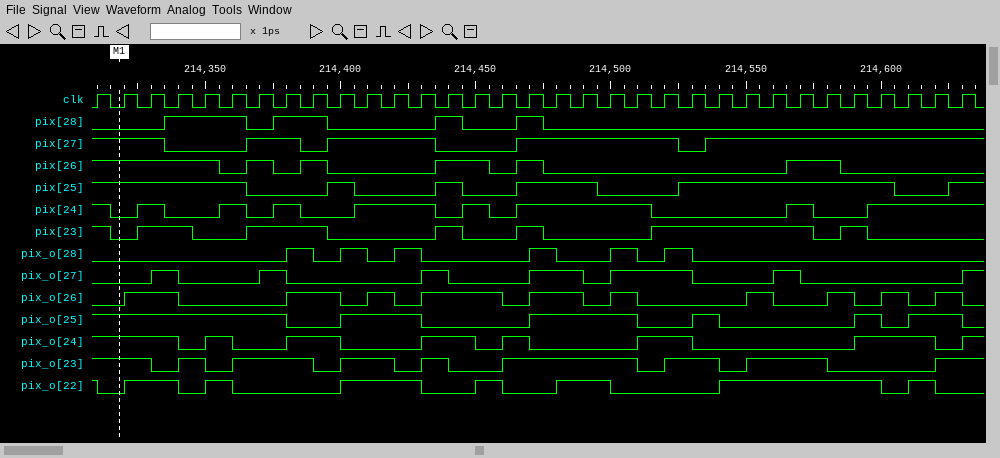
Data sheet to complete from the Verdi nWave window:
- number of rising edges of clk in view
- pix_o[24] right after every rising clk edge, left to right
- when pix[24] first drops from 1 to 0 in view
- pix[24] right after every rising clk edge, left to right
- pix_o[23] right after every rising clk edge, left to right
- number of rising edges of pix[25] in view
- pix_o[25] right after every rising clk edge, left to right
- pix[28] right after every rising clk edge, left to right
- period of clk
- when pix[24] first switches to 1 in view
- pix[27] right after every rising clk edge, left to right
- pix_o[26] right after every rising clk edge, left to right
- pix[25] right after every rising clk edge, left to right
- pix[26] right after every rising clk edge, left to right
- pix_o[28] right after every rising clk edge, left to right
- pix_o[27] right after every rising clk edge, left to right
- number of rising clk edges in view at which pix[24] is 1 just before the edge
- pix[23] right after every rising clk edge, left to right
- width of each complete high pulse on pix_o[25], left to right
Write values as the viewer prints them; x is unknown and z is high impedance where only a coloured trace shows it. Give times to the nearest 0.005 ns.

33
1 1 1 0 1 0 0 1 1 0 0 0 1 1 0 1 0 0 0 0 1 1 0 0 0 0 0 0 1 1 1 0 1
214.315 ns
1 0 1 0 0 1 0 1 0 0 1 1 1 0 1 0 1 1 1 1 1 0 0 0 0 0 1 0 0 1 1 1 1
1 1 0 1 0 1 1 1 0 1 1 0 1 0 0 1 1 1 1 1 0 1 1 0 1 1 1 0 0 0 0 1 1
5
1 1 1 1 1 1 1 0 0 1 1 1 0 0 0 0 1 1 1 1 0 0 1 0 0 0 0 0 1 0 1 1 0
0 0 0 1 1 1 0 1 1 0 0 0 0 1 0 0 1 0 0 0 0 0 0 0 0 0 0 0 0 0 0 0 0
0.01 ns
214.325 ns
1 1 1 0 0 0 1 1 0 1 1 1 1 0 0 0 1 1 1 1 1 1 0 1 1 1 1 1 1 1 1 1 1
0 1 1 0 0 0 0 1 1 0 1 0 1 1 1 0 1 1 0 1 0 0 0 0 1 0 0 1 0 1 0 1 0
1 1 1 1 1 1 0 0 0 1 0 0 0 1 0 0 1 1 1 0 0 0 1 1 1 1 1 1 1 1 0 0 1
1 1 1 1 1 0 1 0 1 0 0 0 0 1 1 0 1 0 0 0 0 0 0 0 0 0 1 1 0 0 0 0 0
0 0 0 0 0 0 0 1 0 1 0 1 0 0 0 0 1 0 0 1 0 1 0 0 0 0 0 0 0 0 0 0 0
0 0 1 0 0 0 1 0 0 0 0 0 1 0 0 0 1 1 0 1 1 1 0 0 0 1 0 0 0 0 0 0 1
18
1 0 1 1 0 0 1 1 1 0 0 0 0 1 0 0 1 0 0 0 0 1 1 1 1 1 1 0 1 0 0 0 0
0.03 ns, 0.04 ns, 0.01 ns, 0.01 ns, 0.02 ns
